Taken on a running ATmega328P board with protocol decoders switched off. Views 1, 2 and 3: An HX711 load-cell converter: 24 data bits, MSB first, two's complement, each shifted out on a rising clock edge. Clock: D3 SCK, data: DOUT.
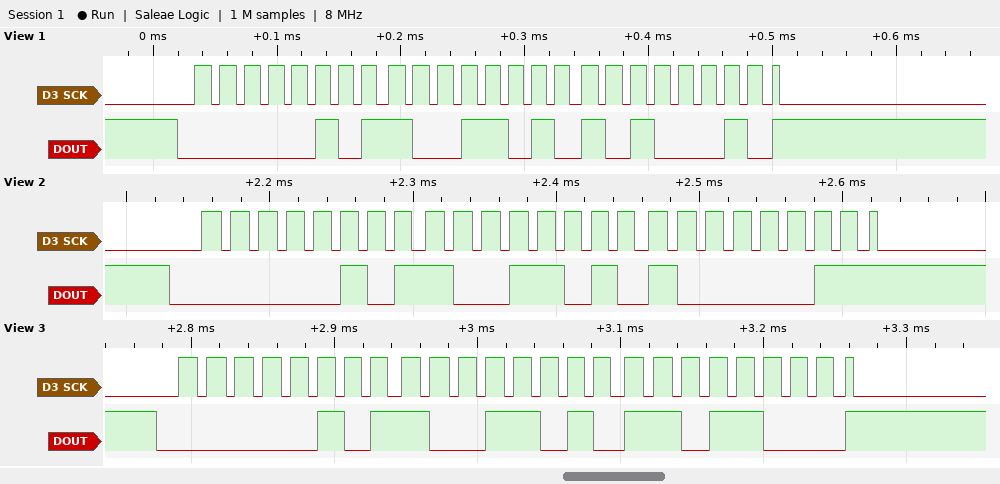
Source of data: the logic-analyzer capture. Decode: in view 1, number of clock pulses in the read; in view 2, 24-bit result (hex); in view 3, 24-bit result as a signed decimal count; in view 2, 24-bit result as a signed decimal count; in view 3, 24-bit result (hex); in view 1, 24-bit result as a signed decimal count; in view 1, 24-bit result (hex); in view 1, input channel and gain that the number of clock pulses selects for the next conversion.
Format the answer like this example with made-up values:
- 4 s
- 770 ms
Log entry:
- 25
- 0x059A83
- 367320
- 367235
- 0x059AD8
- 367266
- 0x059AA2
- channel A, gain 128
